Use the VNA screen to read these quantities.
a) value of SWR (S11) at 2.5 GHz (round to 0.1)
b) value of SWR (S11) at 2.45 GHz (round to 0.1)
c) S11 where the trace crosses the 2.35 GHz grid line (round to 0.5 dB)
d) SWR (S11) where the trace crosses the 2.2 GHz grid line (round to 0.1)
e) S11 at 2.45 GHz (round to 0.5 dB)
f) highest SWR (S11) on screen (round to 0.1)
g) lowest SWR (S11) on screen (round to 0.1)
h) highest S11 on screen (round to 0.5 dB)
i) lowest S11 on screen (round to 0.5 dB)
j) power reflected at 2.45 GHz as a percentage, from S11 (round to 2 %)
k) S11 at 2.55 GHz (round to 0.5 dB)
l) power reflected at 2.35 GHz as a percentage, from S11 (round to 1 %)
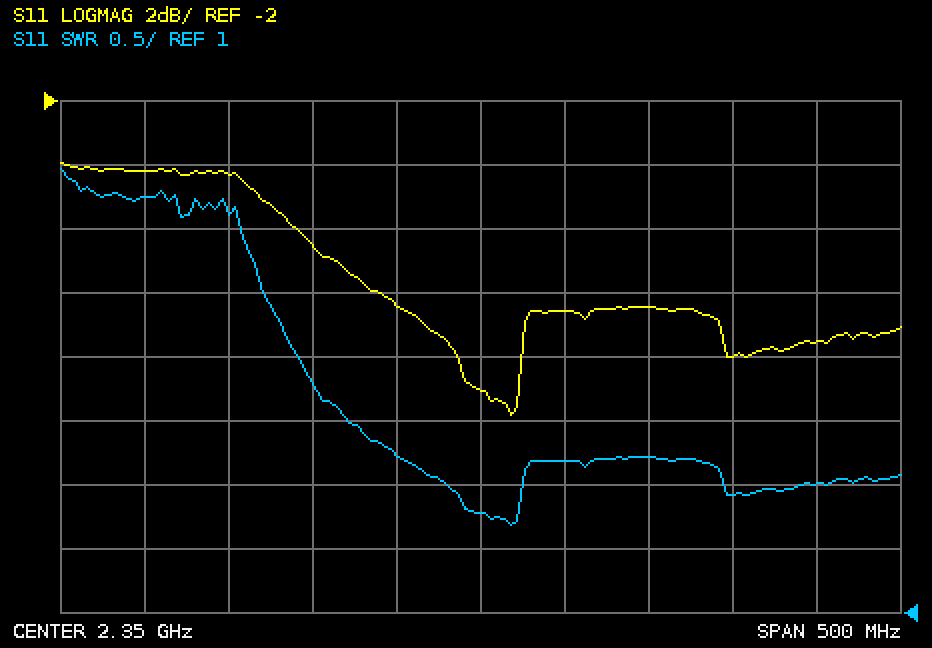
1.9
2.2
-11.0 dB
4.1
-8.5 dB
4.5
1.7
-4.0 dB
-12.0 dB
14 %
-9.5 dB
8 %
